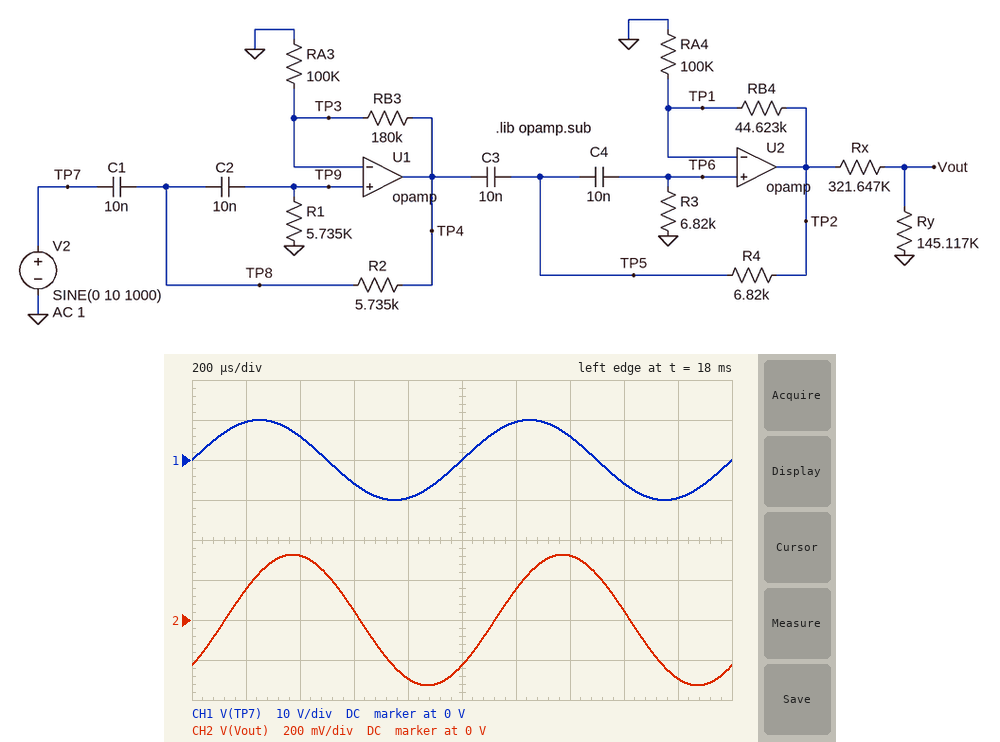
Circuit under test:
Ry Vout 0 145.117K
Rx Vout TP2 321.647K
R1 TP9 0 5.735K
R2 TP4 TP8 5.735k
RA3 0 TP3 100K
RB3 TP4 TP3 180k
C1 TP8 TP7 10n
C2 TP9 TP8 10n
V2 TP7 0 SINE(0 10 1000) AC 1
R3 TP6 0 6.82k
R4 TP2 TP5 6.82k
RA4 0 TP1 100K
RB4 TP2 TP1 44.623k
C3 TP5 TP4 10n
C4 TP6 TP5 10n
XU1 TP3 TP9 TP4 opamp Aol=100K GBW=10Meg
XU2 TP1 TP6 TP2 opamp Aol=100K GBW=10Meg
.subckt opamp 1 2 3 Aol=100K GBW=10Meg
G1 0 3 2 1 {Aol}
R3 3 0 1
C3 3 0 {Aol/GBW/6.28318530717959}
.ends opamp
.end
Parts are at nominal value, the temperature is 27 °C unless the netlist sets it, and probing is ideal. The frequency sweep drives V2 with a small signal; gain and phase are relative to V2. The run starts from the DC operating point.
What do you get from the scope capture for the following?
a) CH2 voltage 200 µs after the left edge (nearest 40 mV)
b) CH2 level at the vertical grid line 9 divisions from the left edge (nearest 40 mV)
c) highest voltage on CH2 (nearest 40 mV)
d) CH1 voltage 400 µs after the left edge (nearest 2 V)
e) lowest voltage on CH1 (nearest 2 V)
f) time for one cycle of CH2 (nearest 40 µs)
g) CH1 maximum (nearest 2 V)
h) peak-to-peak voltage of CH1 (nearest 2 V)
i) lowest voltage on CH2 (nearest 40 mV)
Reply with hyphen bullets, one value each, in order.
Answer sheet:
- 160 mV
- -280 mV
- 320 mV
- 6 V
- -10 V
- 1.00 ms
- 10 V
- 20 V
- -320 mV
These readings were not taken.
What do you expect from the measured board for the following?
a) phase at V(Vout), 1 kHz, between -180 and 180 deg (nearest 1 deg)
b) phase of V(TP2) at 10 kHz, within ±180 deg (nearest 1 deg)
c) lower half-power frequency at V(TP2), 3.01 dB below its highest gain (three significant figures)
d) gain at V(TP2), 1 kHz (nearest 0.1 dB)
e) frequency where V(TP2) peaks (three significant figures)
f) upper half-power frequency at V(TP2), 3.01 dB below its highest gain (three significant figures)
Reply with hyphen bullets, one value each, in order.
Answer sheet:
- -44 deg
- 24 deg
- 2.58 kHz
- -19.6 dB
- 2.82 kHz
- 3.20 kHz
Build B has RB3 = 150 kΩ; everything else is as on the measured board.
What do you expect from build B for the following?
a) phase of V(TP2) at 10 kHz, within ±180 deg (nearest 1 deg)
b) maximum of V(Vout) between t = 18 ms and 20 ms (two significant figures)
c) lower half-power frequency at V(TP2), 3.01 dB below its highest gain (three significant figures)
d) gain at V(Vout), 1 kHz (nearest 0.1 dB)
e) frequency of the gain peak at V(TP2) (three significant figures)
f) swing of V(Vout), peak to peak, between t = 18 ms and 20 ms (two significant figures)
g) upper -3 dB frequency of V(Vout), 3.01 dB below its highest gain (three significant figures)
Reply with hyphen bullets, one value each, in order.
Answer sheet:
- 29 deg
- 290 mV
- 2.51 kHz
- -30.9 dB
- 3.12 kHz
- 570 mV
- 6.21 kHz
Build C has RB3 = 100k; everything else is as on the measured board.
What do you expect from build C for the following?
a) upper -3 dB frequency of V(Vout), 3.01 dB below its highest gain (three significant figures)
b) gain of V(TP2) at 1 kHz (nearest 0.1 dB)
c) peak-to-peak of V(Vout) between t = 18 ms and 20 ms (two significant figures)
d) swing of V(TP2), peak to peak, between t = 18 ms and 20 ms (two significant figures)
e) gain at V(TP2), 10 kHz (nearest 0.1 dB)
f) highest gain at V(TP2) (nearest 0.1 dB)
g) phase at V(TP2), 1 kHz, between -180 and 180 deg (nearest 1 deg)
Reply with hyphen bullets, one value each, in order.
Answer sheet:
- 3.35 MHz
- -23.2 dB
- 430 mV
- 1.4 V
- 9.4 dB
- 9.7 dB
- -62 deg
